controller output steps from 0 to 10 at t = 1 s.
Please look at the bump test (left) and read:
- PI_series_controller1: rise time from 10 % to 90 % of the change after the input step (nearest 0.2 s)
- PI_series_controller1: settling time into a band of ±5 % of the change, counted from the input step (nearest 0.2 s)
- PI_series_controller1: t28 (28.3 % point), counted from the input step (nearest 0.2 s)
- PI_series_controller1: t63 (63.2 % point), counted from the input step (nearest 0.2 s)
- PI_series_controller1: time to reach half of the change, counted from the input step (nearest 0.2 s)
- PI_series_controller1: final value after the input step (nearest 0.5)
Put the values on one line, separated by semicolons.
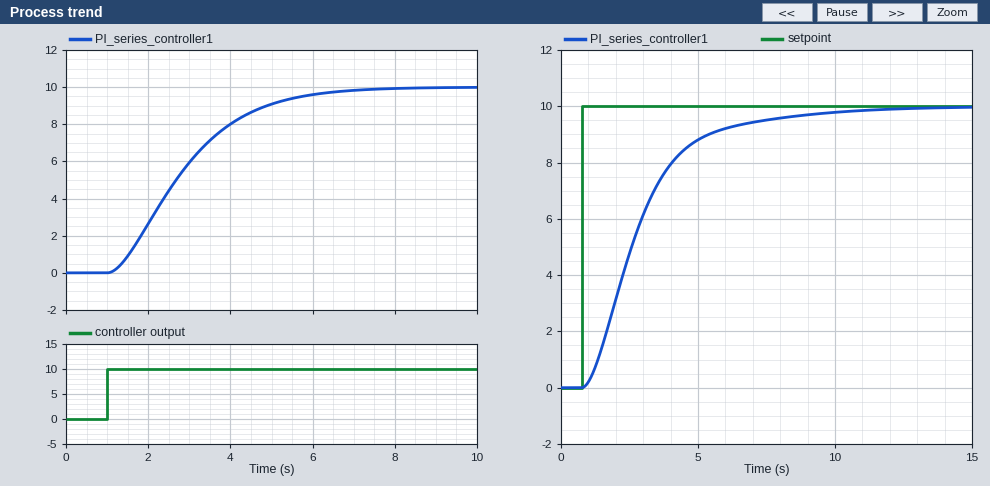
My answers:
3.4 s; 4.8 s; 1.0 s; 2.2 s; 1.6 s; 10.0
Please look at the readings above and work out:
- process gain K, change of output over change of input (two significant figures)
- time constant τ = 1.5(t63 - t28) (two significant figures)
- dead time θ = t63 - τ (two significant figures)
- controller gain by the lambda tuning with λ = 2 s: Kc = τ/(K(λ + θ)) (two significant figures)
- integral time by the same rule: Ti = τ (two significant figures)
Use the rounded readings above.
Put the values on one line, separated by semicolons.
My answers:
1.0; 1.8 s; 0.40 s; 0.75; 1.8 s
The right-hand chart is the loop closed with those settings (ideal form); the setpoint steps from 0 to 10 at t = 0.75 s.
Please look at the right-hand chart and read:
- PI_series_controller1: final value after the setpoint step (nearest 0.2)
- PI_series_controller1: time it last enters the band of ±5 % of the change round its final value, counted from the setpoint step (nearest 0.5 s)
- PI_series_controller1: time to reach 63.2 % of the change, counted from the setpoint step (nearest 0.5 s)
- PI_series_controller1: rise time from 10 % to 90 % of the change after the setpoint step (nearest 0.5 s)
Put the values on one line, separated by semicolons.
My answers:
10.0; 6.5 s; 2.5 s; 4.0 s
